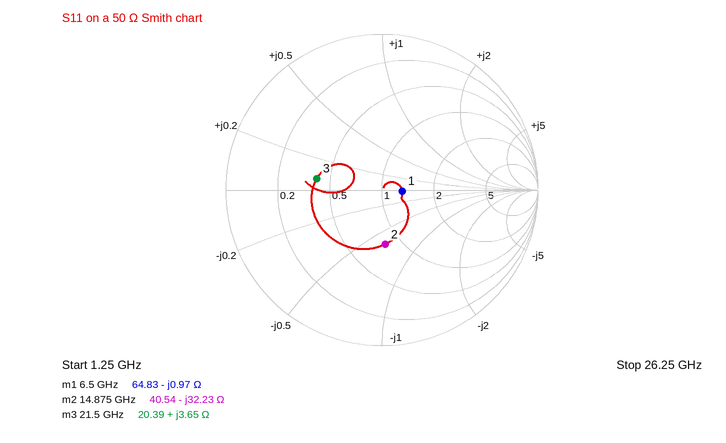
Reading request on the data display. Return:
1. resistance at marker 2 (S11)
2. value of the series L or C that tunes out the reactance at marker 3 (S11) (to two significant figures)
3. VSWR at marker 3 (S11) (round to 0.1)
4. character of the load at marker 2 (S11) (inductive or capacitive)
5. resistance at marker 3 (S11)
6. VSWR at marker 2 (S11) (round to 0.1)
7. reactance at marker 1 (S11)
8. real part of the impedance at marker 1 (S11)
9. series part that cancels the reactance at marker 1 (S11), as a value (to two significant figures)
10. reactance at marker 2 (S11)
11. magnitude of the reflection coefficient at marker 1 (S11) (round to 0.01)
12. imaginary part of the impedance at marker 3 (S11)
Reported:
40.54 Ω
2.0 pF
2.5
capacitive
20.39 Ω
2.1
-0.97 Ω
64.83 Ω
24 pH
-32.23 Ω
0.13
+3.65 Ω
